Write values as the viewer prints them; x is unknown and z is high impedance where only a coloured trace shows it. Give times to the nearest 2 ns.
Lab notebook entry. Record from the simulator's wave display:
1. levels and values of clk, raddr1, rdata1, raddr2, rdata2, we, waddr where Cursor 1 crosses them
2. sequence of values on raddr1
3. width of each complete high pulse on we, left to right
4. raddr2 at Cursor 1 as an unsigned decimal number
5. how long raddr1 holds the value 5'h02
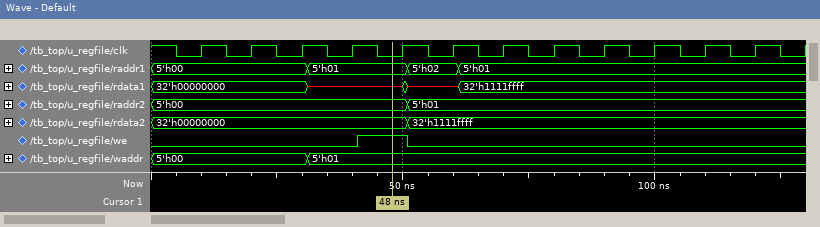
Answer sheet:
clk=0, raddr1=5'h01, rdata1=x, raddr2=5'h00, rdata2=32'h00000000, we=1, waddr=5'h01
5'h00, 5'h01, 5'h02, 5'h01
10 ns
0
10 ns
